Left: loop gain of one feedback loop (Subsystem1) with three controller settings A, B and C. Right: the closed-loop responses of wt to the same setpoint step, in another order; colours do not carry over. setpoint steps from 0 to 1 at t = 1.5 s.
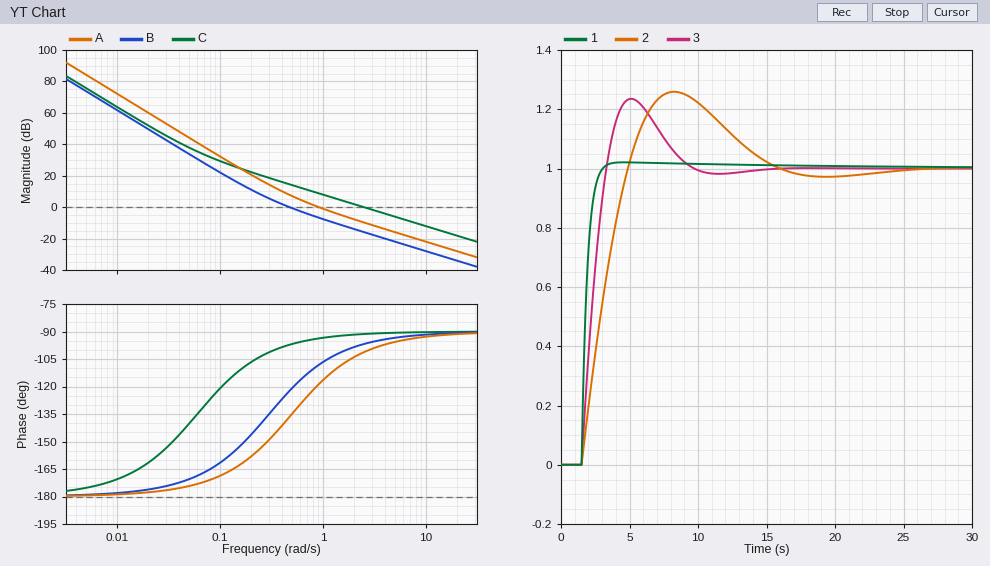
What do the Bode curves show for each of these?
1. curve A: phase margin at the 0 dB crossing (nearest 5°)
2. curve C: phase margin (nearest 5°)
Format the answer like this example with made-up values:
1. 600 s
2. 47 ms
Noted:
1. 60°
2. 90°
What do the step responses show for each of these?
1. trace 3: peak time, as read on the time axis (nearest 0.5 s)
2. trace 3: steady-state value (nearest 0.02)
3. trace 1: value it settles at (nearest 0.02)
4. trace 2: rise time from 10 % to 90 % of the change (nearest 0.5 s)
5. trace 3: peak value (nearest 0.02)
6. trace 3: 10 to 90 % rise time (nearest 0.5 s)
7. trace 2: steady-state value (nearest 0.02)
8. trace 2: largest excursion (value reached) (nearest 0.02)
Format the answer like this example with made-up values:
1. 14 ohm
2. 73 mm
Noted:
1. 5.0 s
2. 1.00
3. 1.00
4. 2.5 s
5. 1.24
6. 1.5 s
7. 1.00
8. 1.26
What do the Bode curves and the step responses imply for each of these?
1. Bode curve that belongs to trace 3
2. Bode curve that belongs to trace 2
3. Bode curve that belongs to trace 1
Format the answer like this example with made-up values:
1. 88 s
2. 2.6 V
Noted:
1. A
2. B
3. C
